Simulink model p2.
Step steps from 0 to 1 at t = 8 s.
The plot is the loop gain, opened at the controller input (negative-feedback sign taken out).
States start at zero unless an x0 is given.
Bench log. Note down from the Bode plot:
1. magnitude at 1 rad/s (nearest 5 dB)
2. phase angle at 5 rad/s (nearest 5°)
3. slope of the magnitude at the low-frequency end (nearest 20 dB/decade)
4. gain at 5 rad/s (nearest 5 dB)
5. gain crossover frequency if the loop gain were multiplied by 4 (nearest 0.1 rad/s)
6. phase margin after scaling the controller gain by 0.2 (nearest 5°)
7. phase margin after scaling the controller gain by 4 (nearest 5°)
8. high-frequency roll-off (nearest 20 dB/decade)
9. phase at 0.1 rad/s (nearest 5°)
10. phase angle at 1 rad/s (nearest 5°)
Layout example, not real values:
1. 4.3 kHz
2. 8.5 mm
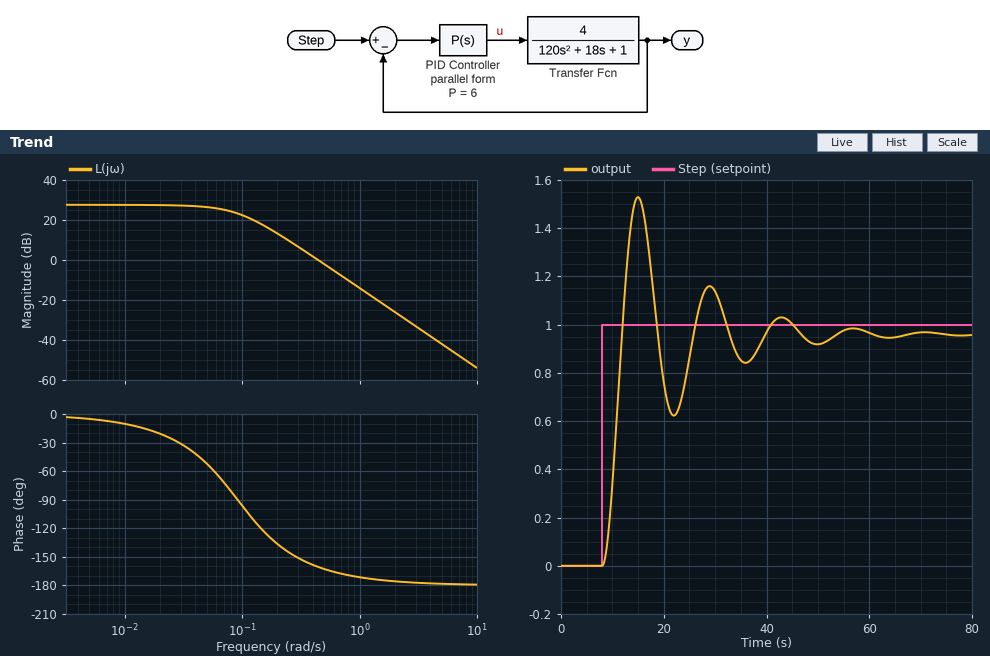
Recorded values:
1. -15 dB
2. -180°
3. 0 dB/decade
4. -40 dB
5. 0.9 rad/s
6. 45°
7. 10°
8. -40 dB/decade
9. -95°
10. -170°
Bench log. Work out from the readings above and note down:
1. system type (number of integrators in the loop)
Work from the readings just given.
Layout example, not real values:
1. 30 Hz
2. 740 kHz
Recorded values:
1. 0
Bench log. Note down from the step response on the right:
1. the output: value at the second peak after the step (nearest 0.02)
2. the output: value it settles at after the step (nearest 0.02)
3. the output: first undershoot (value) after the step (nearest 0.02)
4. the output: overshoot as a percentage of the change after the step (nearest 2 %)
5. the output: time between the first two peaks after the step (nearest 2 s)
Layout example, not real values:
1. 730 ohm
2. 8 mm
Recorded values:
1. 1.16
2. 0.96
3. 0.62
4. 60 %
5. 14 s
